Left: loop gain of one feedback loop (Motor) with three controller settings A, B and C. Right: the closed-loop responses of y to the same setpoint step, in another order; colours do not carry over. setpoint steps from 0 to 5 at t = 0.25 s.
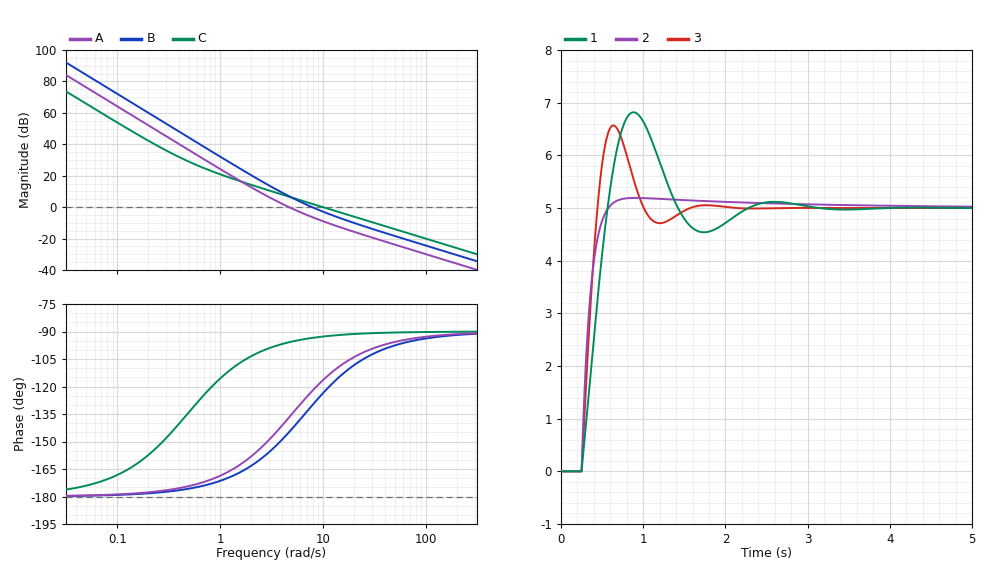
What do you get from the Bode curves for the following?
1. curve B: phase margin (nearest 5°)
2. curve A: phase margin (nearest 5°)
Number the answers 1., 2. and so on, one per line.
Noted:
1. 50°
2. 45°
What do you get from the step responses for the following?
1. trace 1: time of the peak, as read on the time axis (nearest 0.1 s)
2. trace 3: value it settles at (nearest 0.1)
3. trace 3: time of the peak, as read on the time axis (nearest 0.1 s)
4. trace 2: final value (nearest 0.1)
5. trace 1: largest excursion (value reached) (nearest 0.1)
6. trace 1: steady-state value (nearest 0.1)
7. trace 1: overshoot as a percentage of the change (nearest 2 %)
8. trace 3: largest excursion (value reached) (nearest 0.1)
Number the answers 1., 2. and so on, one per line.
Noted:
1. 0.9 s
2. 5.0
3. 0.6 s
4. 5.0
5. 6.8
6. 5.0
7. 36 %
8. 6.6
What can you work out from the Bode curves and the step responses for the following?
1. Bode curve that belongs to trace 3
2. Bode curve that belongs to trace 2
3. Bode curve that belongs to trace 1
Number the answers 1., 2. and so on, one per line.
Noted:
1. B
2. C
3. A
